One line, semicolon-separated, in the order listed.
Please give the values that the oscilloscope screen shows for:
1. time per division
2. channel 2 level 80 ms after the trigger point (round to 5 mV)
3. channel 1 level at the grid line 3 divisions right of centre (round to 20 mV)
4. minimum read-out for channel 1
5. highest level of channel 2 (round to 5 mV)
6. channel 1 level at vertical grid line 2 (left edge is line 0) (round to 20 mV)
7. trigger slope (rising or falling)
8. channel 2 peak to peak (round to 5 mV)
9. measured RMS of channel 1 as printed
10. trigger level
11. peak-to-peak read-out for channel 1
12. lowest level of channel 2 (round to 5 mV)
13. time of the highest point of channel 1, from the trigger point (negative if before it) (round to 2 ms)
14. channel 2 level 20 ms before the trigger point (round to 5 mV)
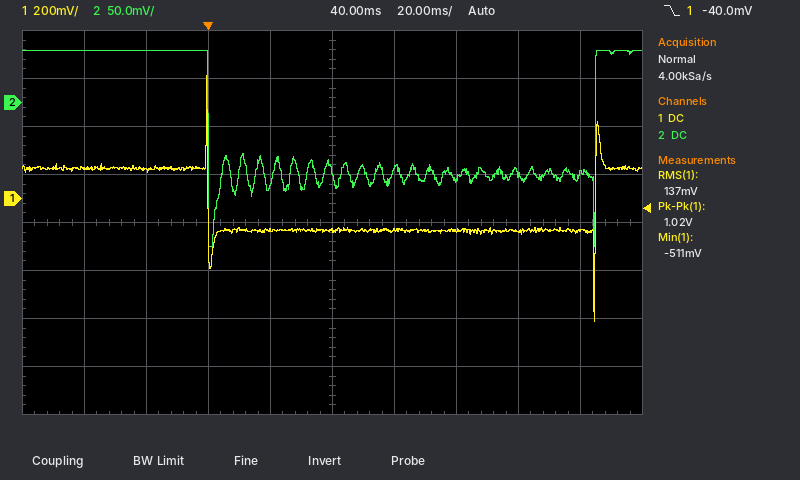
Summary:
20 ms; -80 mV; -140 mV; -511 mV; 55 mV; 120 mV; falling; 205 mV; 137 mV; -40.0 mV; 1.02 V; -150 mV; 0 ms; 55 mV
